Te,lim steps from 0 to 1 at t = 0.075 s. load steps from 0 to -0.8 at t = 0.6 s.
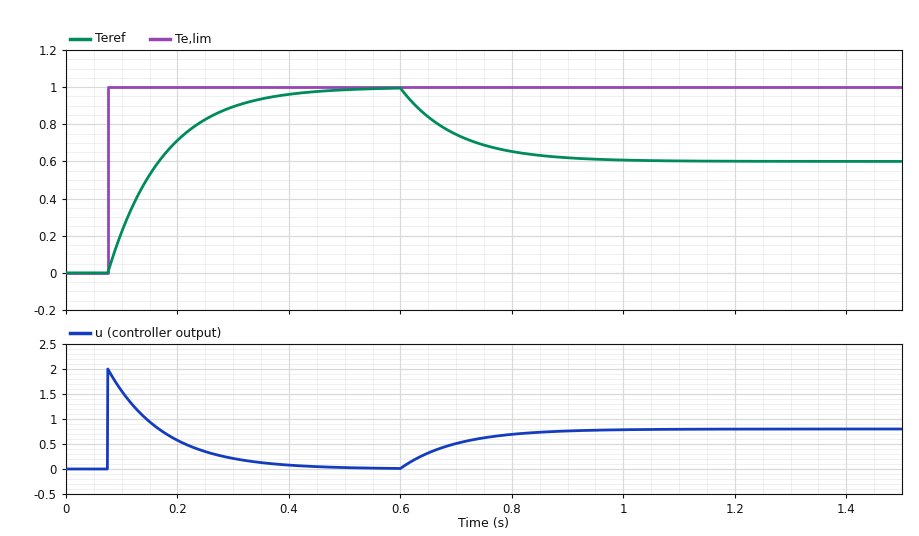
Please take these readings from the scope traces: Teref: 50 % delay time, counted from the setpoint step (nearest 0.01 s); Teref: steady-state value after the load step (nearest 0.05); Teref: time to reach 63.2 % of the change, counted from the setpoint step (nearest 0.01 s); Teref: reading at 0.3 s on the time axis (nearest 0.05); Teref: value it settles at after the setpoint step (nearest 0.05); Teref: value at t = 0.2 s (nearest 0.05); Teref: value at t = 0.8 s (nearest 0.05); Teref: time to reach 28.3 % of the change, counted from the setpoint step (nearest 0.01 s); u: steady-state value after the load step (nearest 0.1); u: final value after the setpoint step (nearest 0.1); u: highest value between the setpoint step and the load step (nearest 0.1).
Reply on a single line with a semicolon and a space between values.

0.07 s; 0.60; 0.10 s; 0.90; 1.00; 0.70; 0.65; 0.03 s; 0.8; 0.0; 2.0
